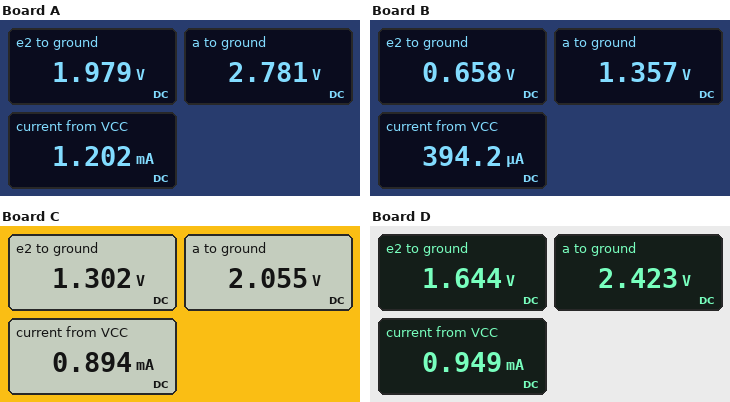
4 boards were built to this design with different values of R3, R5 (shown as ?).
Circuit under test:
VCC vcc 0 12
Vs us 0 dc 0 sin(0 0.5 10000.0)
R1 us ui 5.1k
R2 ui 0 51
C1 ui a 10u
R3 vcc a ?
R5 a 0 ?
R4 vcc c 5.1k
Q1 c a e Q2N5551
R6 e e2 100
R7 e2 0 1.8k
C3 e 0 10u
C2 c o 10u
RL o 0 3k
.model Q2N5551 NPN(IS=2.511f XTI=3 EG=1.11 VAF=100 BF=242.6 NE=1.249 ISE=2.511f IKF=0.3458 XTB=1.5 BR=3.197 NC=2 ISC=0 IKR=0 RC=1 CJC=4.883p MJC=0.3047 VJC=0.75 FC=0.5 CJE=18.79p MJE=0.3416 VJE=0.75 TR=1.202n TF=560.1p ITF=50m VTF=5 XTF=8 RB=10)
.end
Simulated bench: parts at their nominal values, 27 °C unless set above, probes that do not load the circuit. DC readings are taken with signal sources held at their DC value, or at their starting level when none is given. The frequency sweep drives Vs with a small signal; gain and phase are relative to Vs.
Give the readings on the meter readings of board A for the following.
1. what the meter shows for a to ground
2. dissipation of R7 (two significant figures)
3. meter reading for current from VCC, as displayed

2.781 V
2.2 mW
1.202 mA
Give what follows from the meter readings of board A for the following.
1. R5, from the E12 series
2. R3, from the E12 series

27 kΩ
82 kΩ
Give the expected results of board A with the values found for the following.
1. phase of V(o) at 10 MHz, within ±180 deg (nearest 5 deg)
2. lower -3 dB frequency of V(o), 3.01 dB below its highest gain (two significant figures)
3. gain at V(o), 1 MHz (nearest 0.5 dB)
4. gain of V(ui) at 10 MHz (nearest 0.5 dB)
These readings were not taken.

125 deg
660 Hz
-2.5 dB
-43.5 dB
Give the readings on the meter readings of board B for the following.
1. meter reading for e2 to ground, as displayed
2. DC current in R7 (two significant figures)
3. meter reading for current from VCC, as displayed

0.658 V
370 µA
394.2 µA
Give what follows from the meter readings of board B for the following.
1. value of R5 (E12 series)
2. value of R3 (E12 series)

47 kΩ
330 kΩ
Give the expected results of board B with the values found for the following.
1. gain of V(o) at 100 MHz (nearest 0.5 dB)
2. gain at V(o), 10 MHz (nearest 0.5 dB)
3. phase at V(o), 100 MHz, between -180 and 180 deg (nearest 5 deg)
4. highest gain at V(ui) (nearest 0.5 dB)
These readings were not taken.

-28.5 dB
-13.0 dB
60 deg
-40.0 dB
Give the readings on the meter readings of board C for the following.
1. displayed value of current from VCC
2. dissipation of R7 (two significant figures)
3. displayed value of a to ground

0.894 mA
940 µW
2.055 V
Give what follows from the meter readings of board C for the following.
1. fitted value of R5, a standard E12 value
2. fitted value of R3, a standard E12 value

12 kΩ
56 kΩ
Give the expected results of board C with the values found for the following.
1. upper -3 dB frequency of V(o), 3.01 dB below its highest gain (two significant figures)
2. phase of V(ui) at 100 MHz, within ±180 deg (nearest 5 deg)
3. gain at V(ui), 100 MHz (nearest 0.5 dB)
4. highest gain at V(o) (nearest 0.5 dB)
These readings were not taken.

11 MHz
-25 deg
-48.5 dB
-6.0 dB
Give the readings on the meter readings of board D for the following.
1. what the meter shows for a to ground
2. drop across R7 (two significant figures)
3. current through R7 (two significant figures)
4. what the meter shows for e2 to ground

2.423 V
1.6 V
910 µA
1.644 V
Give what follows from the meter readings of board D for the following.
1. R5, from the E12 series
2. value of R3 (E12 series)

68 kΩ
220 kΩ
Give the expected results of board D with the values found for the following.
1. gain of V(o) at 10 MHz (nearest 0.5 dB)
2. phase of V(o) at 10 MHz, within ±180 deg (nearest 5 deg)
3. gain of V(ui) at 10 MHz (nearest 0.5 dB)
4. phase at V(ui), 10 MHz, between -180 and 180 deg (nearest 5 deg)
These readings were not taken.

-7.5 dB
130 deg
-43.0 dB
-25 deg
